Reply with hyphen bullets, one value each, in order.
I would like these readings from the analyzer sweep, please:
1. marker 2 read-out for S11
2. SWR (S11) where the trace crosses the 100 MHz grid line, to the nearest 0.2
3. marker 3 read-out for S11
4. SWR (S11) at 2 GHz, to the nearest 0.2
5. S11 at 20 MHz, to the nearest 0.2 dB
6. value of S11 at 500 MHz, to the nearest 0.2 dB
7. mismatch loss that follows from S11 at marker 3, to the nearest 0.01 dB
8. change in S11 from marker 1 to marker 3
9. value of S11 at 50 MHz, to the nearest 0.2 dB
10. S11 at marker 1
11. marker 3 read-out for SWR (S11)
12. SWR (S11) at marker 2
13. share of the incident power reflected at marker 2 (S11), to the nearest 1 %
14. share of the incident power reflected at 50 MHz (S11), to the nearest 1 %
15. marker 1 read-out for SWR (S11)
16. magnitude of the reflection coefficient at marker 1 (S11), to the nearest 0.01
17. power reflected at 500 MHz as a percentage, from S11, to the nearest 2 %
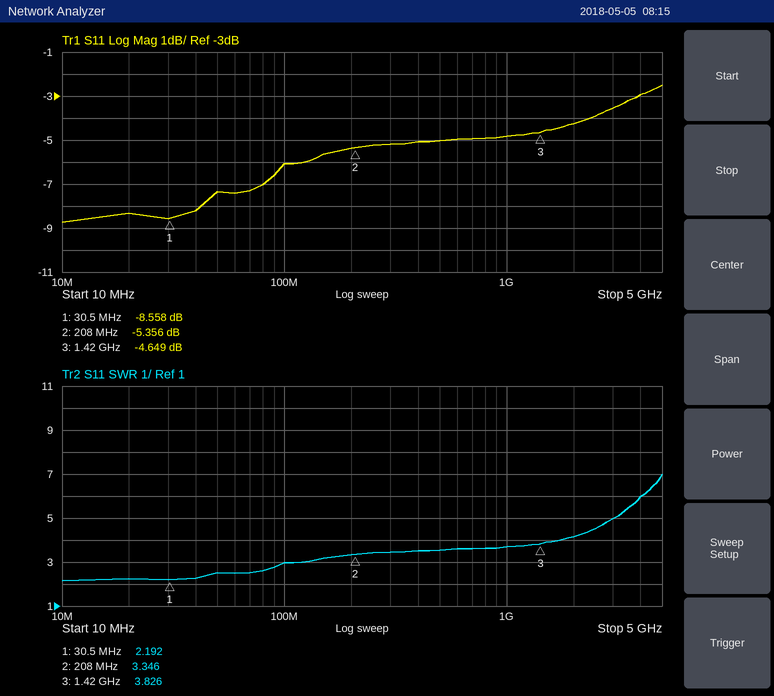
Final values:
- -5.356 dB
- 3.0
- -4.649 dB
- 4.2
- -8.4 dB
- -5.0 dB
- 1.82 dB
- 3.909 dB
- -7.4 dB
- -8.558 dB
- 3.826
- 3.346
- 29 %
- 18 %
- 2.192
- 0.37
- 32 %
